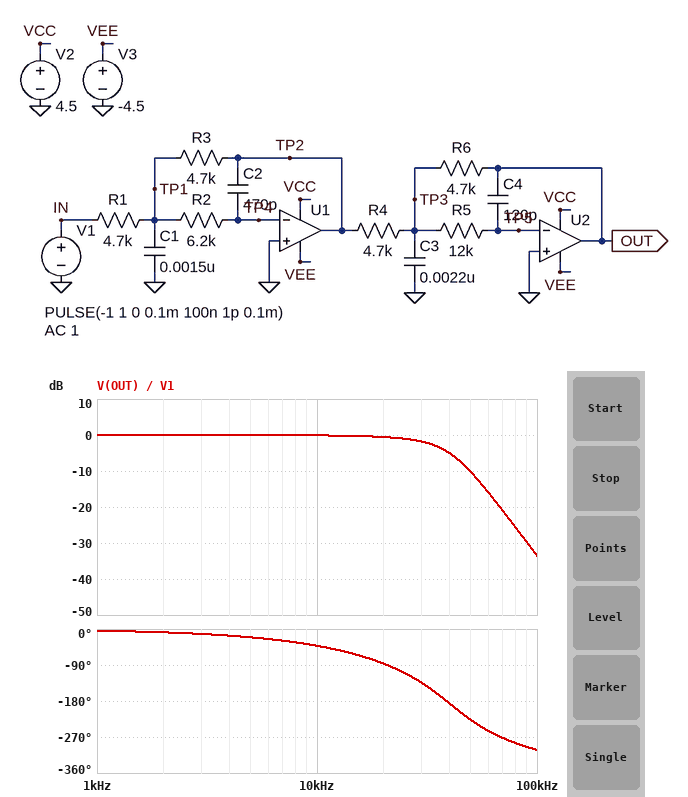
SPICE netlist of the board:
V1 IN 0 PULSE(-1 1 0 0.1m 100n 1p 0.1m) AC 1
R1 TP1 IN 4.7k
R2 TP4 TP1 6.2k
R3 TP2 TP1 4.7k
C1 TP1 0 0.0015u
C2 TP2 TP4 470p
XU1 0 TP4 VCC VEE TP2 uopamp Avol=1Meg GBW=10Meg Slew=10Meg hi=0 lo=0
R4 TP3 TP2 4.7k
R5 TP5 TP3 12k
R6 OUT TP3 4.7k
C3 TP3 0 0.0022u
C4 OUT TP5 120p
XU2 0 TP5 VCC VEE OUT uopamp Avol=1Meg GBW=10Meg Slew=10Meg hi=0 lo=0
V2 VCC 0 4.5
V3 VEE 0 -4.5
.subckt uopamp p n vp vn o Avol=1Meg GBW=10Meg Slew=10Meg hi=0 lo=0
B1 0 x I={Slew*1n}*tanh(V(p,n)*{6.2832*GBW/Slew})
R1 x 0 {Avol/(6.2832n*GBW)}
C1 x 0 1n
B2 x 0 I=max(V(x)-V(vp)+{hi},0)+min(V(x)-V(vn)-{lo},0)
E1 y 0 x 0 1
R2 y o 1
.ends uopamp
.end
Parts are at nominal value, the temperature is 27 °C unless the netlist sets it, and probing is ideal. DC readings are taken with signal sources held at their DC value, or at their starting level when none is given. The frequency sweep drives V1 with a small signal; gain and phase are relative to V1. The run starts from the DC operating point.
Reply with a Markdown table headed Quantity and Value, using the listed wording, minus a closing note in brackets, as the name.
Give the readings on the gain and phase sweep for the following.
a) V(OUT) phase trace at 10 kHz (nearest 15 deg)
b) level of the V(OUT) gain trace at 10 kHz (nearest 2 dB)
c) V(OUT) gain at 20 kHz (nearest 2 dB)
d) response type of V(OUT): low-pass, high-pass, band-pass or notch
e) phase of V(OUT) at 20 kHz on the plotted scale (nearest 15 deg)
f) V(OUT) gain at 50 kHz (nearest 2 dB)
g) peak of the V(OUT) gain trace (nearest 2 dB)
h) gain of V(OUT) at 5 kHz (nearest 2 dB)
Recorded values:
| Quantity | Value |
|---|---|
| V(OUT) phase trace at 10 kHz | -45 deg |
| level of the V(OUT) gain trace at 10 kHz | 0 dB |
| V(OUT) gain at 20 kHz | 0 dB |
| response type of V(OUT): low-pass, high-pass, band-pass or notch | low-pass |
| phase of V(OUT) at 20 kHz on the plotted scale | -90 deg |
| V(OUT) gain at 50 kHz | -10 dB |
| peak of the V(OUT) gain trace | 0 dB |
| gain of V(OUT) at 5 kHz | 0 dB |
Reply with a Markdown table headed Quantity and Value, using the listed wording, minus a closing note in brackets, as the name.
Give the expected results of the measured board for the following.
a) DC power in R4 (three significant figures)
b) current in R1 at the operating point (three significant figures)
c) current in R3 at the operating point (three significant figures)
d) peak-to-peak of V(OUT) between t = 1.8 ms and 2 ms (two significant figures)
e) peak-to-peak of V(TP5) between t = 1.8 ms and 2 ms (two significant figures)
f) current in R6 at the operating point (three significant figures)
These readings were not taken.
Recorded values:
| Quantity | Value |
|---|---|
| DC power in R4 | 213 µW |
| current in R1 at the operating point | 213 µA |
| current in R3 at the operating point | 213 µA |
| peak-to-peak of V(OUT) between t = 1.8 ms and 2 ms | 1.7 V |
| peak-to-peak of V(TP5) between t = 1.8 ms and 2 ms | 3.0 mV |
| current in R6 at the operating point | 213 µA |
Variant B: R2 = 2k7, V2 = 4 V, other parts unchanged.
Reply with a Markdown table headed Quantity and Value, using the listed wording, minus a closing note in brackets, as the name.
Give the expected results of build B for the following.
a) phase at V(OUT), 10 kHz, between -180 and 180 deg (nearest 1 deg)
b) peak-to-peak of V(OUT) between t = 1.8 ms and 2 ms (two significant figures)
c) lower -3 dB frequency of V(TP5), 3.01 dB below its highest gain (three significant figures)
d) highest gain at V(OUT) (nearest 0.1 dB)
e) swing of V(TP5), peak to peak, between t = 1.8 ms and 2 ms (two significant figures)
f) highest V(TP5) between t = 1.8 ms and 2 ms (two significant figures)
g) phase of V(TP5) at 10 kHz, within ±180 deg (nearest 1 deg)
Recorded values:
| Quantity | Value |
|---|---|
| phase at V(OUT), 10 kHz, between -180 and 180 deg | -30 deg |
| peak-to-peak of V(OUT) between t = 1.8 ms and 2 ms | 2.0 V |
| lower -3 dB frequency of V(TP5), 3.01 dB below its highest gain | 23.4 kHz |
| highest gain at V(OUT) | 1.0 dB |
| swing of V(TP5), peak to peak, between t = 1.8 ms and 2 ms | 4.4 mV |
| highest V(TP5) between t = 1.8 ms and 2 ms | 3.3 mV |
| phase of V(TP5) at 10 kHz, within ±180 deg | -120 deg |
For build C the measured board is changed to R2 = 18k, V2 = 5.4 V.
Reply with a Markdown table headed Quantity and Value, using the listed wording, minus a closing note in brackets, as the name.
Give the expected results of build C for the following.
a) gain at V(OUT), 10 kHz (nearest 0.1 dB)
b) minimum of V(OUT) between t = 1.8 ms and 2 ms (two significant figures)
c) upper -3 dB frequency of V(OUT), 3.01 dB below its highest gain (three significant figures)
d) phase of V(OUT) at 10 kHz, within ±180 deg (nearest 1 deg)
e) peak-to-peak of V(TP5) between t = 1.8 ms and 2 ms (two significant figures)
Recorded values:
| Quantity | Value |
|---|---|
| gain at V(OUT), 10 kHz | -2.8 dB |
| minimum of V(OUT) between t = 1.8 ms and 2 ms | -430 mV |
| upper -3 dB frequency of V(OUT), 3.01 dB below its highest gain | 10.6 kHz |
| phase of V(OUT) at 10 kHz, within ±180 deg | -71 deg |
| peak-to-peak of V(TP5) between t = 1.8 ms and 2 ms | 1.5 mV |
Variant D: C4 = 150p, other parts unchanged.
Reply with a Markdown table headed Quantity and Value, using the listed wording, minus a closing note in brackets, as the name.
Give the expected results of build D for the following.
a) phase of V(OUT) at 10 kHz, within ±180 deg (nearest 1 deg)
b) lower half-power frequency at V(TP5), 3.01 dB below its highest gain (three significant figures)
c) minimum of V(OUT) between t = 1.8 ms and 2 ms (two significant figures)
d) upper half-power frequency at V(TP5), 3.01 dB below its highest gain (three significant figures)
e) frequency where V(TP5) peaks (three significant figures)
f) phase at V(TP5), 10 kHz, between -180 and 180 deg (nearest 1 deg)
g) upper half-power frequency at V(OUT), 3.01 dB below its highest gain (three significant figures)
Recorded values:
| Quantity | Value |
|---|---|
| phase of V(OUT) at 10 kHz, within ±180 deg | -45 deg |
| lower half-power frequency at V(TP5), 3.01 dB below its highest gain | 16.3 kHz |
| minimum of V(OUT) between t = 1.8 ms and 2 ms | -870 mV |
| upper half-power frequency at V(TP5), 3.01 dB below its highest gain | 43.1 kHz |
| frequency where V(TP5) peaks | 29.3 kHz |
| phase at V(TP5), 10 kHz, between -180 and 180 deg | -135 deg |
| upper half-power frequency at V(OUT), 3.01 dB below its highest gain | 31.1 kHz |
